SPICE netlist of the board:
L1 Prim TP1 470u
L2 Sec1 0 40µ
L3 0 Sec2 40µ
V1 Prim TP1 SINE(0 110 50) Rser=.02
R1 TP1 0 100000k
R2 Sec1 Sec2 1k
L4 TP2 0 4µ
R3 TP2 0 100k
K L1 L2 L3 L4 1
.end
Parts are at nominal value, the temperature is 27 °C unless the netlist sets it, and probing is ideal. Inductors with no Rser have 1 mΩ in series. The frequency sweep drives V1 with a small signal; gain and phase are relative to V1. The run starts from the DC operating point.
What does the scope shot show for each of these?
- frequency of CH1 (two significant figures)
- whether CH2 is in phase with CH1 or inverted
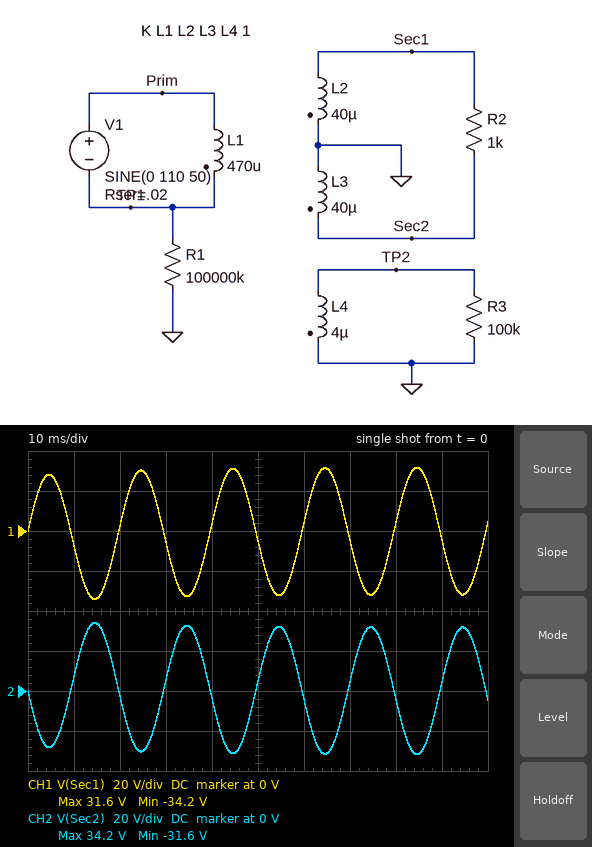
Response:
50 Hz
inverted
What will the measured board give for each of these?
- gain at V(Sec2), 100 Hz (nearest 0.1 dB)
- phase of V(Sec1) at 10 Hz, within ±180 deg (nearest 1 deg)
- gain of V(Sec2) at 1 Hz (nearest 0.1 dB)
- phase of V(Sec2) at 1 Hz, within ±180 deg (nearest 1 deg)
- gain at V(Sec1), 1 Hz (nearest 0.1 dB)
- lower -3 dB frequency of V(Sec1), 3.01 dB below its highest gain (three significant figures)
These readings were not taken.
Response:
-10.7 dB
35 deg
-27.8 dB
-98 deg
-27.8 dB
7.11 Hz
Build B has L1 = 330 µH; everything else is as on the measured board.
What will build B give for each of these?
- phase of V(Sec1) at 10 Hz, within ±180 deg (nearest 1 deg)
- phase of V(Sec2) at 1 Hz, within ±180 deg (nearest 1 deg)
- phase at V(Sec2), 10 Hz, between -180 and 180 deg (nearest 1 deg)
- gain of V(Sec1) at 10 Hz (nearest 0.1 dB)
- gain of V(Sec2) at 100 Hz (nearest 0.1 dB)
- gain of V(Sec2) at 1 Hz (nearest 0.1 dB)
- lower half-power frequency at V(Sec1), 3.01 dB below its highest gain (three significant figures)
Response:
45 deg
-96 deg
-135 deg
-12.2 dB
-9.2 dB
-29.3 dB
10.1 Hz
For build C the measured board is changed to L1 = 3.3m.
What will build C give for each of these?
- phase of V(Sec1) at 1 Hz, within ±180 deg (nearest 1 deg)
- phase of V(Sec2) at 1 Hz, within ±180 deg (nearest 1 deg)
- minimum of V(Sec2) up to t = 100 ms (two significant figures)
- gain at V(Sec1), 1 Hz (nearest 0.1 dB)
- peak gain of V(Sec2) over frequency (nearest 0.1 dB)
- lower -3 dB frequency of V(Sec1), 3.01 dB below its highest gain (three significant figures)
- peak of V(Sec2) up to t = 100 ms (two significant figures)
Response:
45 deg
-135 deg
-12 V
-22.2 dB
-19.2 dB
1.01 Hz
12 V
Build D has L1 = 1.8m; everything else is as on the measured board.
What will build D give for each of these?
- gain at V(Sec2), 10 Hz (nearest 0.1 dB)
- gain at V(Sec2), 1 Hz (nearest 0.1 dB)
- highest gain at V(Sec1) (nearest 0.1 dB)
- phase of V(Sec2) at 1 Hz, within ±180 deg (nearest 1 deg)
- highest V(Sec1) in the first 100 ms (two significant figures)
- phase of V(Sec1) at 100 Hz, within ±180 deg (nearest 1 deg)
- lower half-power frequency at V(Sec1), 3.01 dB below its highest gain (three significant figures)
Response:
-16.7 dB
-23.0 dB
-16.5 dB
-118 deg
16 V
1 deg
1.86 Hz
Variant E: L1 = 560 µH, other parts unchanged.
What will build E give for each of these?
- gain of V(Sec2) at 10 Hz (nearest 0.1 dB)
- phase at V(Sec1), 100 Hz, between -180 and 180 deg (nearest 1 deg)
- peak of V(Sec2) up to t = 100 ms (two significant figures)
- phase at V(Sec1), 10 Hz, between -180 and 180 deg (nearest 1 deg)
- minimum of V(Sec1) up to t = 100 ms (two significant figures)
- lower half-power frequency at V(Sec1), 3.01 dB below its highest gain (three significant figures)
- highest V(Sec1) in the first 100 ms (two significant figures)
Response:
-12.8 dB
3 deg
31 V
31 deg
-31 V
5.97 Hz
29 V
